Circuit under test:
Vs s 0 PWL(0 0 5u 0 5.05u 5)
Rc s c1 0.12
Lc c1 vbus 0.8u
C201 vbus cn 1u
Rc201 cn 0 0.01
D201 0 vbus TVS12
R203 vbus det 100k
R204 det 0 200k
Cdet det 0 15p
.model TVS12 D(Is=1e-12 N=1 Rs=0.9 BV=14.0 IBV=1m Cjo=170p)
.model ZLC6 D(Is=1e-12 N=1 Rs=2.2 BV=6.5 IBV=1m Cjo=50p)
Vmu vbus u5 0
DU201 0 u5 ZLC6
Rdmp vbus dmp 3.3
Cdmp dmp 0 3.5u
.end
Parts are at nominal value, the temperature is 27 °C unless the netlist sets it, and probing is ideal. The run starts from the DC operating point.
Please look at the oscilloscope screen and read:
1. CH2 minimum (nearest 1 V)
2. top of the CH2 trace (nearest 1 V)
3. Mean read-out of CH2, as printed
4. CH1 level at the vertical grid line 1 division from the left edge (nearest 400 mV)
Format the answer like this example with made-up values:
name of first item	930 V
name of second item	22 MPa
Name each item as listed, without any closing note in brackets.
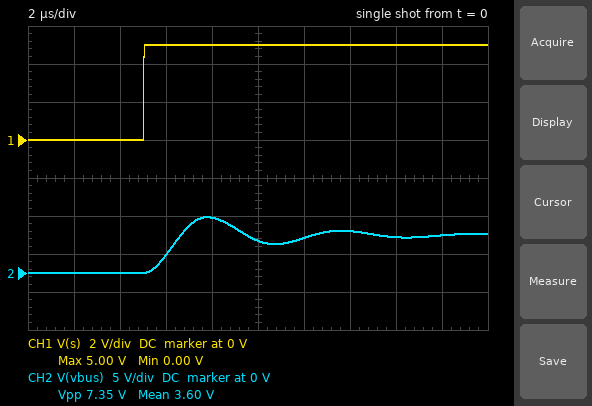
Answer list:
CH2 minimum	0 V
top of the CH2 trace	7 V
Mean read-out of CH2, as printed	3.60 V
CH1 level at the vertical grid line 1 division from the left edge	0 V
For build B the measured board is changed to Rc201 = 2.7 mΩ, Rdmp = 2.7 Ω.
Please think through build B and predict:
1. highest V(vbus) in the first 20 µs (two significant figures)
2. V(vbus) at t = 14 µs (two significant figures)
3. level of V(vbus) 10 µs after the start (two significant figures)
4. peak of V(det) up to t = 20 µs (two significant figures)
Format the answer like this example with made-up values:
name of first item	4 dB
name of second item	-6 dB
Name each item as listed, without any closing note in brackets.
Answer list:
highest V(vbus) in the first 20 µs	7.2 V
V(vbus) at t = 14 µs	5.4 V
level of V(vbus) 10 µs after the start	4.4 V
peak of V(det) up to t = 20 µs	4.1 V
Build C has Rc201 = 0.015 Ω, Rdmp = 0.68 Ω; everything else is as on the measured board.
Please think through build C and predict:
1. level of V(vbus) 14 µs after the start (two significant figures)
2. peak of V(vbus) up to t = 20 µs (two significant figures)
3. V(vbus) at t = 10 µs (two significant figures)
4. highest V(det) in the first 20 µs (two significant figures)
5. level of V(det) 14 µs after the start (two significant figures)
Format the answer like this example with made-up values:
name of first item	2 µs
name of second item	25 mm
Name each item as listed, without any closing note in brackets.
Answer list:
level of V(vbus) 14 µs after the start	5.0 V
peak of V(vbus) up to t = 20 µs	6.1 V
V(vbus) at t = 10 µs	6.0 V
highest V(det) in the first 20 µs	3.9 V
level of V(det) 14 µs after the start	3.4 V
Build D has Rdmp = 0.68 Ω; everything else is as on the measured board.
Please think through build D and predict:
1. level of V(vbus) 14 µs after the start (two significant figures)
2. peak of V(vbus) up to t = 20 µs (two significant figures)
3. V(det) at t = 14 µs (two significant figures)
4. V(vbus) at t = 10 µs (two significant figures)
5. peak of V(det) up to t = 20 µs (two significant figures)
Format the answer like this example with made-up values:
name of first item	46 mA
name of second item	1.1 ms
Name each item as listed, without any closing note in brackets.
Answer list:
level of V(vbus) 14 µs after the start	5.0 V
peak of V(vbus) up to t = 20 µs	6.1 V
V(det) at t = 14 µs	3.4 V
V(vbus) at t = 10 µs	6.0 V
peak of V(det) up to t = 20 µs	3.9 V
